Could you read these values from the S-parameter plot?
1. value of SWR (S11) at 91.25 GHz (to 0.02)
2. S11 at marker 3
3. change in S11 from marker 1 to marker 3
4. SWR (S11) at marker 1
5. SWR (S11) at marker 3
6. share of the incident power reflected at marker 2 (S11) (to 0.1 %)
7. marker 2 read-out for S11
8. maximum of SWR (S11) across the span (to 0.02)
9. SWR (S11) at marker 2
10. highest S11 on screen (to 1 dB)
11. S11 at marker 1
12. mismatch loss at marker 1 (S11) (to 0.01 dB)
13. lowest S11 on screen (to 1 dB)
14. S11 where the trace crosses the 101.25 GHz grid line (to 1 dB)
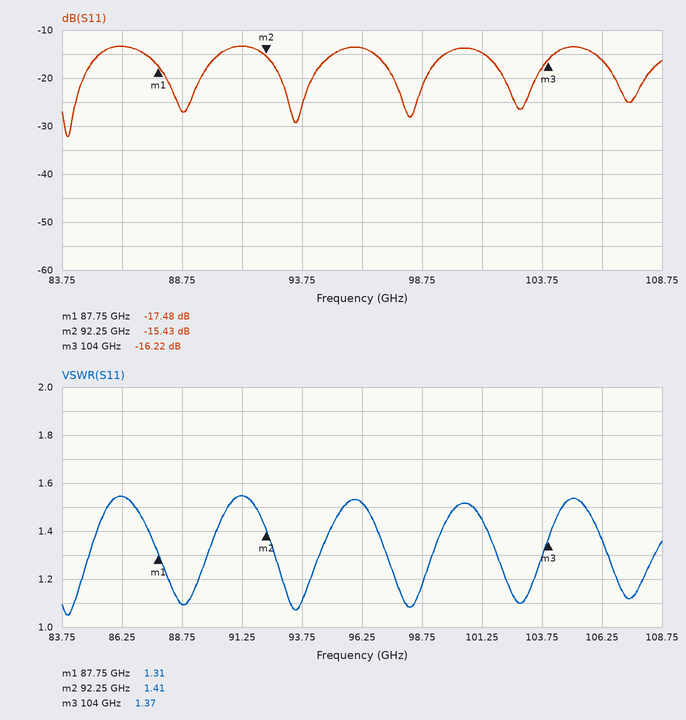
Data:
1.54
-16.22 dB
1.26 dB
1.31
1.37
2.9 %
-15.43 dB
1.54
1.41
-13 dB
-17.48 dB
0.08 dB
-32 dB
-15 dB
